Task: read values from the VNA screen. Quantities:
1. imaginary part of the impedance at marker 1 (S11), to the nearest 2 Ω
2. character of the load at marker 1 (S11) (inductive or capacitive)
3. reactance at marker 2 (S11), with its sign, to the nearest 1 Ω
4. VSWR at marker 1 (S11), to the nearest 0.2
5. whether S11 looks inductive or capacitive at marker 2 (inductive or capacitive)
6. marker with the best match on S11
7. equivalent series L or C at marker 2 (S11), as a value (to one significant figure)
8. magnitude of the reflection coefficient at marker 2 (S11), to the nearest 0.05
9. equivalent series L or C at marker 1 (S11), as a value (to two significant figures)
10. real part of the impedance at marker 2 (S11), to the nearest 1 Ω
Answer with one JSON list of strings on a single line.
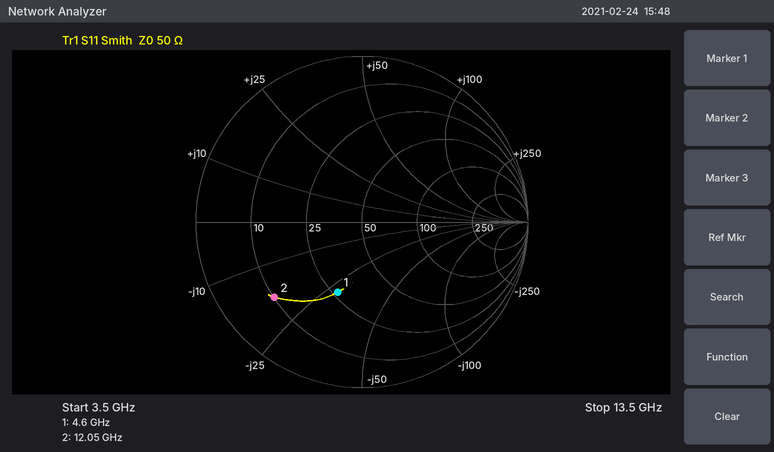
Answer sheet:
["-28 Ω", "capacitive", "-18 Ω", "2.6", "capacitive", "marker 1", "700 fF", "0.70", "1.2 pF", "10 Ω"]
